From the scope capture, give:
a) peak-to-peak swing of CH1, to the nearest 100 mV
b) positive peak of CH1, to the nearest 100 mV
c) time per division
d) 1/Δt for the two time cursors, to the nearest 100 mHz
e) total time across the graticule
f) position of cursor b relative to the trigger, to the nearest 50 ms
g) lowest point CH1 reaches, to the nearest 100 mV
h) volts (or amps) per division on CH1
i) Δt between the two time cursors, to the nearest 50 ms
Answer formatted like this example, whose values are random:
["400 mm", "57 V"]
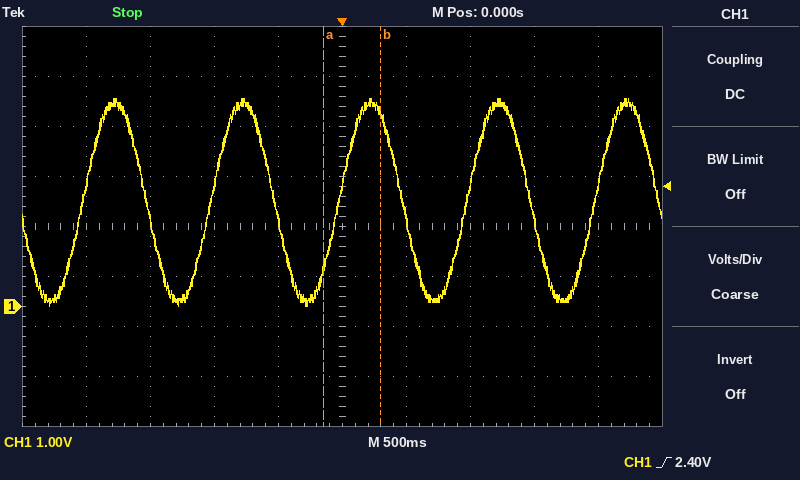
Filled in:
["4.2 V", "4.2 V", "500 ms", "2.2 Hz", "5 s", "+300 ms", "0.0 V", "1 V", "450 ms"]
